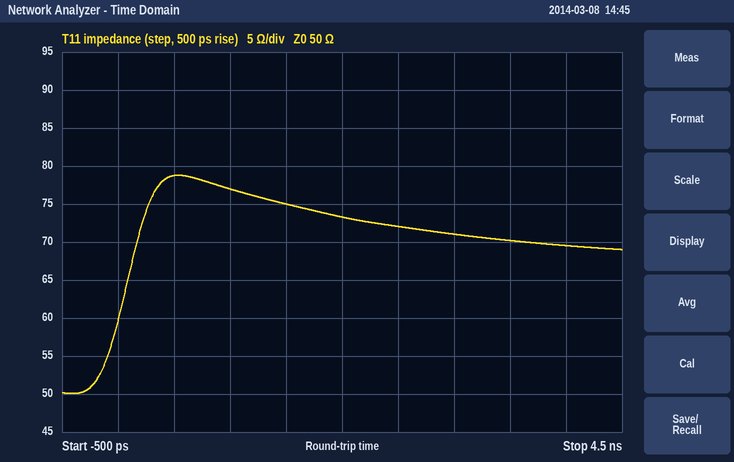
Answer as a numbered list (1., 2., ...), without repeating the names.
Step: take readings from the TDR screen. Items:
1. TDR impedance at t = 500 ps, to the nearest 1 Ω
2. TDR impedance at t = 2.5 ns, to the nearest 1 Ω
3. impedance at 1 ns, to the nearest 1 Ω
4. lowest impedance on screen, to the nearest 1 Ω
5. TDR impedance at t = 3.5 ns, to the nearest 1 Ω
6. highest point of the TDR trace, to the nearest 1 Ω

1. 79 Ω
2. 72 Ω
3. 77 Ω
4. 50 Ω
5. 70 Ω
6. 79 Ω
